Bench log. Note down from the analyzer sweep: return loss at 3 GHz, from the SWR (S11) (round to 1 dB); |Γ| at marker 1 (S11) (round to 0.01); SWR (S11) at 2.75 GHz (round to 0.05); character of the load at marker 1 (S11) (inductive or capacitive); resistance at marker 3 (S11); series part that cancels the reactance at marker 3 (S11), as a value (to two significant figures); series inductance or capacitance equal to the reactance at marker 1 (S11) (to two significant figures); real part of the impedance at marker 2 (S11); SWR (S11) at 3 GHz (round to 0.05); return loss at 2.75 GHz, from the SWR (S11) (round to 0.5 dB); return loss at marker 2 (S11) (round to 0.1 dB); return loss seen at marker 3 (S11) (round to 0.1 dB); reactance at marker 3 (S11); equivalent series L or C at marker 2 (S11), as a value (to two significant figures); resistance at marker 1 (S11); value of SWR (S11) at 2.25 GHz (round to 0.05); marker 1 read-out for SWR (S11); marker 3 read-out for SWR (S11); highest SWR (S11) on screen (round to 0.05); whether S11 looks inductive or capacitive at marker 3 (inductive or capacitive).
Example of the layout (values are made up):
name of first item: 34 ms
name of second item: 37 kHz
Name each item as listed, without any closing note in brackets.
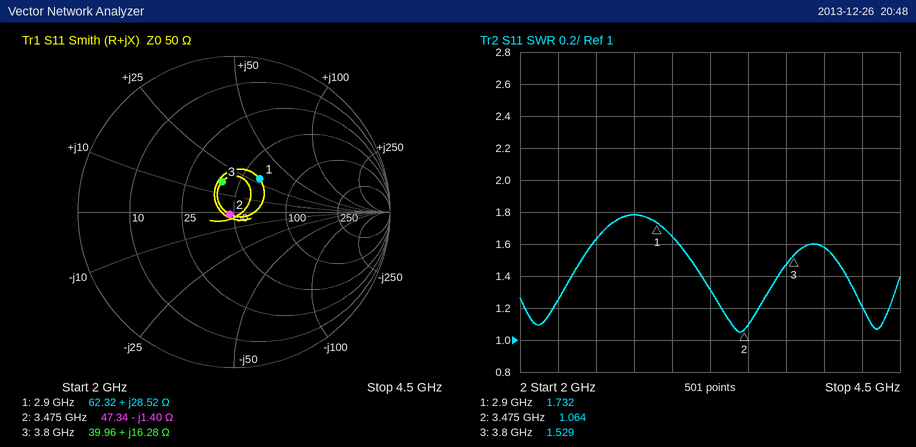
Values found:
return loss at 3 GHz, from the SWR (S11): 12 dB
|Γ| at marker 1 (S11): 0.27
SWR (S11) at 2.75 GHz: 1.80
character of the load at marker 1 (S11): inductive
resistance at marker 3: 39.96 Ω
series part that cancels the reactance at marker 3 (S11), as a value: 2.6 pF
series inductance or capacitance equal to the reactance at marker 1 (S11): 1.6 nH
real part of the impedance at marker 2: 47.34 Ω
SWR (S11) at 3 GHz: 1.65
return loss at 2.75 GHz, from the SWR (S11): 11.0 dB
return loss at marker 2 (S11): 30.2 dB
return loss seen at marker 3 (S11): 13.6 dB
reactance at marker 3: +16.28 Ω
equivalent series L or C at marker 2 (S11), as a value: 33 pF
resistance at marker 1: 62.32 Ω
value of SWR (S11) at 2.25 GHz: 1.25
marker 1 read-out for SWR: 1.732
marker 3 read-out for SWR: 1.529
highest SWR (S11) on screen: 1.80
whether S11 looks inductive or capacitive at marker 3: inductive
